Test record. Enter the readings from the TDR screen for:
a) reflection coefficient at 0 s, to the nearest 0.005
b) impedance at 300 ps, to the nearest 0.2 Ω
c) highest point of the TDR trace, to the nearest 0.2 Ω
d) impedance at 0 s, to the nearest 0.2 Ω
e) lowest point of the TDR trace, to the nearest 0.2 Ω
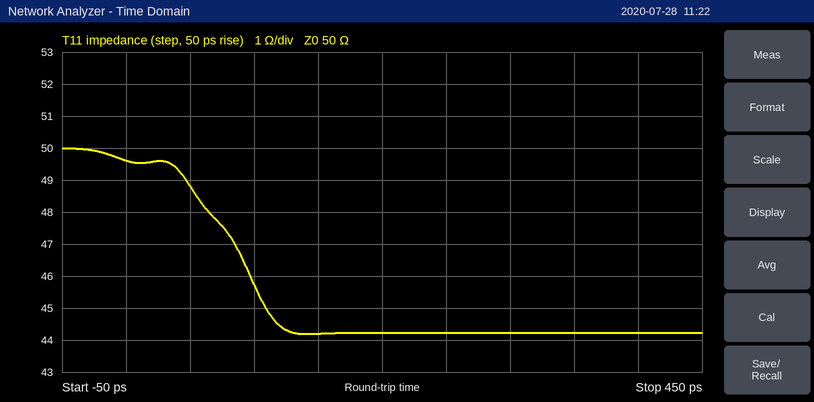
-0.005
44.2 Ω
50.0 Ω
49.6 Ω
44.2 Ω
